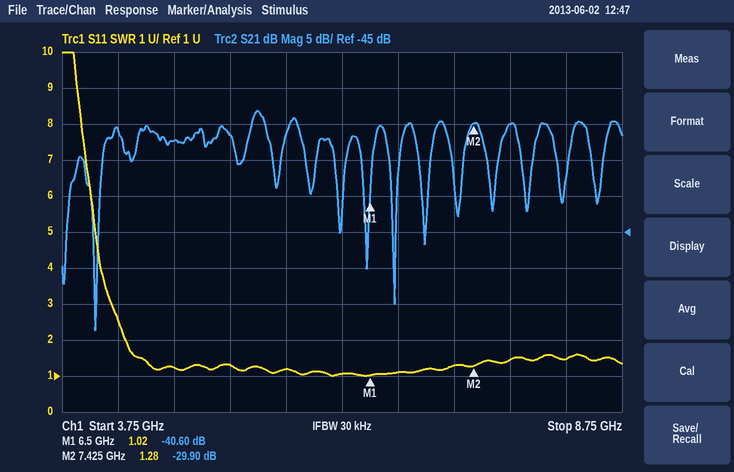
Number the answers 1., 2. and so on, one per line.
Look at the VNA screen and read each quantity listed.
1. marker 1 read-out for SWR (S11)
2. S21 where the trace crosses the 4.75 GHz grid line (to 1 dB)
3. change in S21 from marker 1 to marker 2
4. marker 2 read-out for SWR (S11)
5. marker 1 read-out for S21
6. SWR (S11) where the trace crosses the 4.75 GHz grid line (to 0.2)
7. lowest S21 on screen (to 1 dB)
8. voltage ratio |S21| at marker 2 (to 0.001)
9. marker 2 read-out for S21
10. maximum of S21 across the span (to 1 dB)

1. 1.02
2. -32 dB
3. 10.70 dB
4. 1.28
5. -40.60 dB
6. 1.2
7. -59 dB
8. 0.032
9. -29.90 dB
10. -28 dB
